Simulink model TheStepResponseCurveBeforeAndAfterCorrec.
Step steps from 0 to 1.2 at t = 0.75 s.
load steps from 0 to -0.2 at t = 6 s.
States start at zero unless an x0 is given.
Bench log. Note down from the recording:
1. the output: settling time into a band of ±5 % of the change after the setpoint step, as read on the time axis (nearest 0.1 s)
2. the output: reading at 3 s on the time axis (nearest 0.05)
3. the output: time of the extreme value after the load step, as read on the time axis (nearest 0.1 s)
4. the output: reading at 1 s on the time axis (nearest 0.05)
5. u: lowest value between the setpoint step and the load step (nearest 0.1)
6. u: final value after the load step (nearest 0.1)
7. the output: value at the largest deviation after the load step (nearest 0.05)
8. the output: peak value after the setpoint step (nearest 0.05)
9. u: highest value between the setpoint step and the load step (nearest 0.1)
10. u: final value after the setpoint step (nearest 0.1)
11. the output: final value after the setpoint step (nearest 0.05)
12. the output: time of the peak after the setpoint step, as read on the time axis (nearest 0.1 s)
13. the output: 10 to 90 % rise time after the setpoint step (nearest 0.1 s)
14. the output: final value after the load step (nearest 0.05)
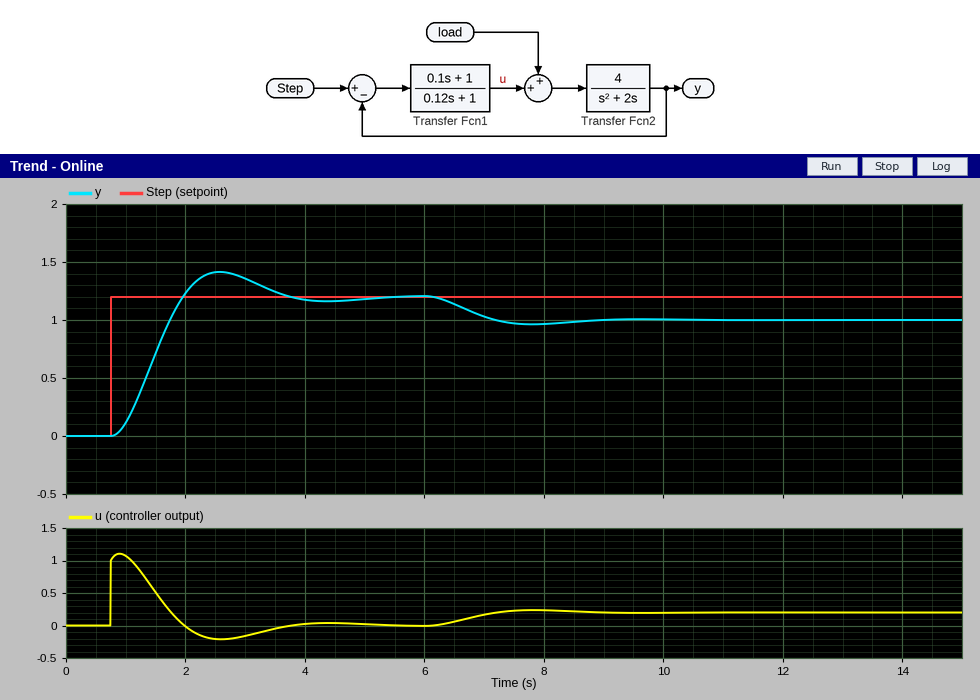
3.4 s
1.35
7.8 s
0.10
-0.2
0.2
0.95
1.40
1.1
0.0
1.20
2.6 s
0.8 s
1.00
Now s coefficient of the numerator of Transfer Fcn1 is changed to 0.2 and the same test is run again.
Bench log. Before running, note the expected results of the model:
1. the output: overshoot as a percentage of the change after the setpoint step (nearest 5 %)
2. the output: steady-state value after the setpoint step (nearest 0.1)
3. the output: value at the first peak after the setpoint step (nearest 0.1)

10 %
1.2
1.3
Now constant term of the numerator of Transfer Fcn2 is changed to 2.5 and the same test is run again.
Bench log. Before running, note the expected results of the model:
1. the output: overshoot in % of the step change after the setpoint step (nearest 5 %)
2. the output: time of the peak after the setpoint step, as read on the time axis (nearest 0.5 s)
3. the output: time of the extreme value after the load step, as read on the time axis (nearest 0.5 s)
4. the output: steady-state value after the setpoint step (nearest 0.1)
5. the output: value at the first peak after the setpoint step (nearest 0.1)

10 %
3.5 s
8.5 s
1.2
1.3
